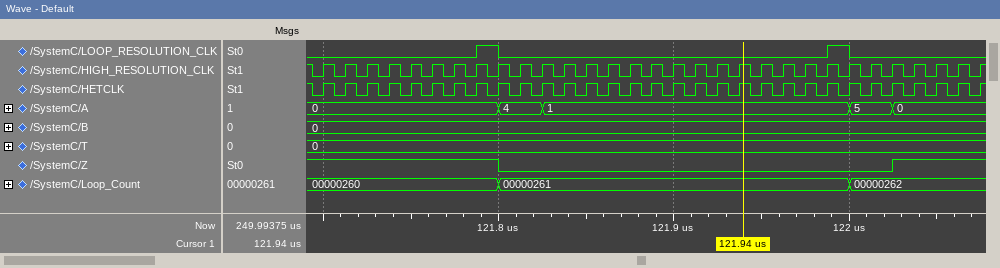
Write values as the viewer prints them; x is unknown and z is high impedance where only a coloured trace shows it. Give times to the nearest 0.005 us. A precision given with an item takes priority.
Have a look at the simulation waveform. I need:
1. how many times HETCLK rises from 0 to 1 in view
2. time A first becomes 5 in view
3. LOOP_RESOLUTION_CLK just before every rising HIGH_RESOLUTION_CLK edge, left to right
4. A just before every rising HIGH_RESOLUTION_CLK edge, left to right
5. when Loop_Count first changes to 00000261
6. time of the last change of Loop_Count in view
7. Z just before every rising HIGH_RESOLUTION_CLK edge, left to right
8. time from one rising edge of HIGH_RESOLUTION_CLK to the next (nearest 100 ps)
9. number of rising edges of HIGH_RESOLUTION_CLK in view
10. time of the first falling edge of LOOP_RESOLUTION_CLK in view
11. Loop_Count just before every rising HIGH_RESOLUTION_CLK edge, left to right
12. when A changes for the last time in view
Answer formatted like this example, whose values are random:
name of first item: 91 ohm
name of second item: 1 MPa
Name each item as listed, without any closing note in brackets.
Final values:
how many times HETCLK rises from 0 to 1 in view: 31
time A first becomes 5 in view: 122 us
LOOP_RESOLUTION_CLK just before every rising HIGH_RESOLUTION_CLK edge, left to right: 0 0 0 0 0 0 0 0 1 0 0 0 0 0 0 0 0 0 0 0 0 0 0 0 1 0 0 0 0 0 0
A just before every rising HIGH_RESOLUTION_CLK edge, left to right: 0, 0, 0, 0, 0, 0, 0, 0, 0, 4, 4, 1, 1, 1, 1, 1, 1, 1, 1, 1, 1, 1, 1, 1, 1, 5, 5, 0, 0, 0, 0
when Loop_Count first changes to 00000261: 121.8 us
time of the last change of Loop_Count in view: 122 us
Z just before every rising HIGH_RESOLUTION_CLK edge, left to right: 1 1 1 1 1 1 1 1 1 0 0 0 0 0 0 0 0 0 0 0 0 0 0 0 0 0 0 1 1 1 1
time from one rising edge of HIGH_RESOLUTION_CLK to the next: 12500 ps
number of rising edges of HIGH_RESOLUTION_CLK in view: 31
time of the first falling edge of LOOP_RESOLUTION_CLK in view: 121.8 us
Loop_Count just before every rising HIGH_RESOLUTION_CLK edge, left to right: 00000260, 00000260, 00000260, 00000260, 00000260, 00000260, 00000260, 00000260, 00000260, 00000261, 00000261, 00000261, 00000261, 00000261, 00000261, 00000261, 00000261, 00000261, 00000261, 00000261, 00000261, 00000261, 00000261, 00000261, 00000261, 00000262, 00000262, 00000262, 00000262, 00000262, 00000262
when A changes for the last time in view: 122.025 us
